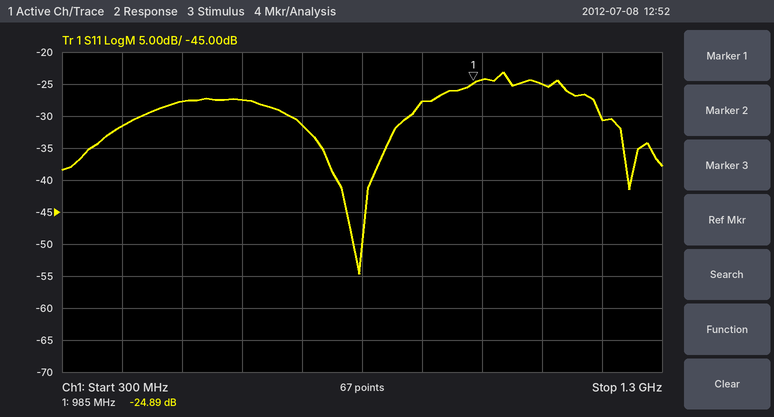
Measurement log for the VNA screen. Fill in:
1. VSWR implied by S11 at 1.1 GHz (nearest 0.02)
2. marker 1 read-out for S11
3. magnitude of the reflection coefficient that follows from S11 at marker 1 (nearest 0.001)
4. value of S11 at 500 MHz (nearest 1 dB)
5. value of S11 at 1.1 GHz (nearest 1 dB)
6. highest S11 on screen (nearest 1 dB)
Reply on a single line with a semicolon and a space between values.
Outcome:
1.12; -24.89 dB; 0.057; -28 dB; -25 dB; -23 dB
